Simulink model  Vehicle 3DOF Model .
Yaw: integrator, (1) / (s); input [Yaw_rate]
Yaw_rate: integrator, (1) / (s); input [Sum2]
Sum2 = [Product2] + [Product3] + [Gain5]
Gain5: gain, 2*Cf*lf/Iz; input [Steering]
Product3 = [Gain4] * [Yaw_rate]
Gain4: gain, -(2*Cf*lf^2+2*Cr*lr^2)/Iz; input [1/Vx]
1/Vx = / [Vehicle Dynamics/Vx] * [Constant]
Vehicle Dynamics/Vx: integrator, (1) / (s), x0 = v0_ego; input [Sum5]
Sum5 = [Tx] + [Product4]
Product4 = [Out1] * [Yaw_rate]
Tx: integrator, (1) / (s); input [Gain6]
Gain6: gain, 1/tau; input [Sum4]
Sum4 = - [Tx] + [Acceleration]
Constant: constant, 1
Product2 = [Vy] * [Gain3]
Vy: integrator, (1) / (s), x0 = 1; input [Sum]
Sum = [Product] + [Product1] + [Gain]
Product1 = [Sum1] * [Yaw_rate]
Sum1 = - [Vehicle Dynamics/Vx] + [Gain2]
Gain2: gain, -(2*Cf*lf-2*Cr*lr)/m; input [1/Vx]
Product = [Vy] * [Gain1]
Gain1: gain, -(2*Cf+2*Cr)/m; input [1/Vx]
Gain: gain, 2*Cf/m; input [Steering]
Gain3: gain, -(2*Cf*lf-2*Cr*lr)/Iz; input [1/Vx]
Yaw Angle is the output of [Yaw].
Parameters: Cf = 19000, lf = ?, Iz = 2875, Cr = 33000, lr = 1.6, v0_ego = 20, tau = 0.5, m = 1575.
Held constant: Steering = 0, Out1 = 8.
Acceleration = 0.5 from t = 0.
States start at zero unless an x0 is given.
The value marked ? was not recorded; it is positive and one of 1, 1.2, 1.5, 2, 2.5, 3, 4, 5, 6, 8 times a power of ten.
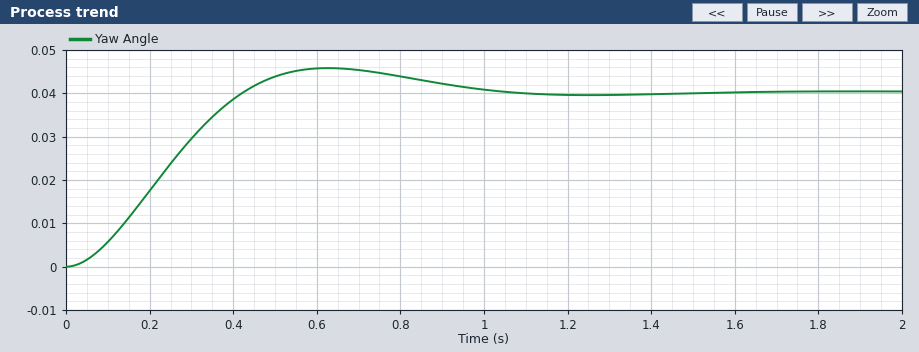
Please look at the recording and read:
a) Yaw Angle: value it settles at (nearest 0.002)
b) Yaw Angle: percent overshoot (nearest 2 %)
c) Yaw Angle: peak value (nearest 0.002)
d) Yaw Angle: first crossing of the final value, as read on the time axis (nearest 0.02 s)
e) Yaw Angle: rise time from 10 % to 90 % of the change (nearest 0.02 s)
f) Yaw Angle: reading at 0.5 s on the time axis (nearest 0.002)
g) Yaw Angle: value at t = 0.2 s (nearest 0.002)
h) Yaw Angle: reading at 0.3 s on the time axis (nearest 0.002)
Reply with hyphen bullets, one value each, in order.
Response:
- 0.040
- 14 %
- 0.046
- 0.42 s
- 0.28 s
- 0.044
- 0.018
- 0.030
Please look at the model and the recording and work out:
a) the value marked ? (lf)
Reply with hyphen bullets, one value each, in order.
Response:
- 0.6
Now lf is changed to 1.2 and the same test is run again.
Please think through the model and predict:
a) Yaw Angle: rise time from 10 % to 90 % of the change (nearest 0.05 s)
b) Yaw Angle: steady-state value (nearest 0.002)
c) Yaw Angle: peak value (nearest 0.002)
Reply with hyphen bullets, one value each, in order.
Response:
- 0.35 s
- 0.032
- 0.036
